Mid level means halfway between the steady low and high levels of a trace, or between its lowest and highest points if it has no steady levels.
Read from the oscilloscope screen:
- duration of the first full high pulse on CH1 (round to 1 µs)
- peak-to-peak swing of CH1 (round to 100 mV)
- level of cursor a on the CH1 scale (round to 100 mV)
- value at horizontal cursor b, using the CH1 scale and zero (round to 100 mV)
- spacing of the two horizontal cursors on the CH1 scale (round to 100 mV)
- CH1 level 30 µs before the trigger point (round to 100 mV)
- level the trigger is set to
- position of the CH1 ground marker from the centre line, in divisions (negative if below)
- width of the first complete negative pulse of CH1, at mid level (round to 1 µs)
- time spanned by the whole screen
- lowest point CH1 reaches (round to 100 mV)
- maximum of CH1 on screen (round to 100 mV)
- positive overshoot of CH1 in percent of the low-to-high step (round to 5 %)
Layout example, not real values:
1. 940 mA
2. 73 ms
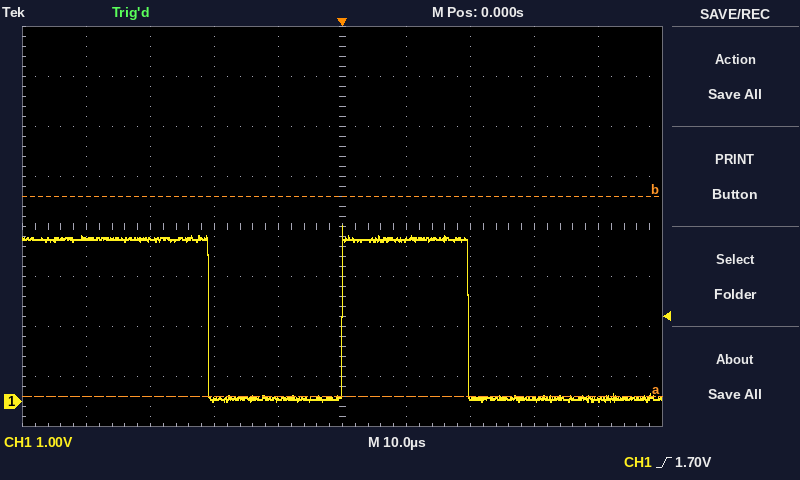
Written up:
1. 20 µs
2. 3.5 V
3. 100 mV
4. 4.1 V
5. 4.0 V
6. 3.2 V
7. 1.70 V
8. -3.5 div
9. 21 µs
10. 100 µs
11. 0.0 V
12. 3.5 V
13. 10 %
